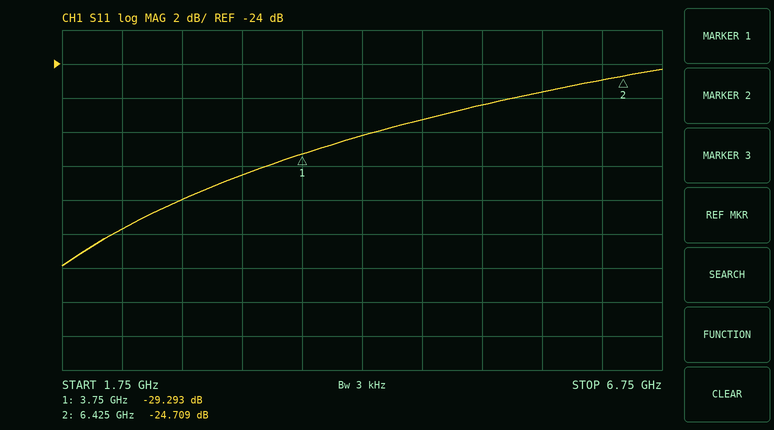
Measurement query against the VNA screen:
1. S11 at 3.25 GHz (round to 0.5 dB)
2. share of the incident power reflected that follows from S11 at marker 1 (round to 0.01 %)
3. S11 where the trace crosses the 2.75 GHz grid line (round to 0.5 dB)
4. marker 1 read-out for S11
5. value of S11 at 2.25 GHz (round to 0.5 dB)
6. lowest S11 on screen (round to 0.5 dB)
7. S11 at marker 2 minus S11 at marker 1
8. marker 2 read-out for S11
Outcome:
-30.5 dB
0.12 %
-32.0 dB
-29.293 dB
-33.5 dB
-36.0 dB
4.584 dB
-24.709 dB
